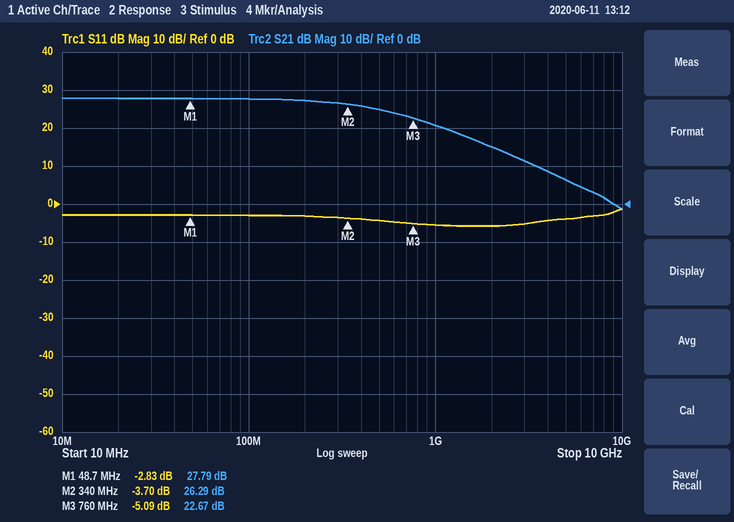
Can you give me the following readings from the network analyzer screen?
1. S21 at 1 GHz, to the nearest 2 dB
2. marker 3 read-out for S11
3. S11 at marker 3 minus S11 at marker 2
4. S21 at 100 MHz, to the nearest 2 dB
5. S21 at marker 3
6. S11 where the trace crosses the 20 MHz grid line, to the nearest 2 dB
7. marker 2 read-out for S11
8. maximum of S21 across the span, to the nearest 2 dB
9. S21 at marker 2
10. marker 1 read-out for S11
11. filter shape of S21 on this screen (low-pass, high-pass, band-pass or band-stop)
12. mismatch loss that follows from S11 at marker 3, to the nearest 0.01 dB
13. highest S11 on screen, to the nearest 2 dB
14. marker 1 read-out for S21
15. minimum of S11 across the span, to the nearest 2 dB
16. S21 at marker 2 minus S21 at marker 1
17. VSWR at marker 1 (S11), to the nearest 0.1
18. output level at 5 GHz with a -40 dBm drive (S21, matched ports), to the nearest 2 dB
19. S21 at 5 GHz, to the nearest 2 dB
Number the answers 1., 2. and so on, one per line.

1. 20 dB
2. -5.09 dB
3. -1.39 dB
4. 28 dB
5. 22.67 dB
6. -2 dB
7. -3.70 dB
8. 28 dB
9. 26.29 dB
10. -2.83 dB
11. low-pass
12. 1.61 dB
13. -2 dB
14. 27.79 dB
15. -6 dB
16. -1.50 dB
17. 6.2
18. -34 dBm
19. 6 dB
